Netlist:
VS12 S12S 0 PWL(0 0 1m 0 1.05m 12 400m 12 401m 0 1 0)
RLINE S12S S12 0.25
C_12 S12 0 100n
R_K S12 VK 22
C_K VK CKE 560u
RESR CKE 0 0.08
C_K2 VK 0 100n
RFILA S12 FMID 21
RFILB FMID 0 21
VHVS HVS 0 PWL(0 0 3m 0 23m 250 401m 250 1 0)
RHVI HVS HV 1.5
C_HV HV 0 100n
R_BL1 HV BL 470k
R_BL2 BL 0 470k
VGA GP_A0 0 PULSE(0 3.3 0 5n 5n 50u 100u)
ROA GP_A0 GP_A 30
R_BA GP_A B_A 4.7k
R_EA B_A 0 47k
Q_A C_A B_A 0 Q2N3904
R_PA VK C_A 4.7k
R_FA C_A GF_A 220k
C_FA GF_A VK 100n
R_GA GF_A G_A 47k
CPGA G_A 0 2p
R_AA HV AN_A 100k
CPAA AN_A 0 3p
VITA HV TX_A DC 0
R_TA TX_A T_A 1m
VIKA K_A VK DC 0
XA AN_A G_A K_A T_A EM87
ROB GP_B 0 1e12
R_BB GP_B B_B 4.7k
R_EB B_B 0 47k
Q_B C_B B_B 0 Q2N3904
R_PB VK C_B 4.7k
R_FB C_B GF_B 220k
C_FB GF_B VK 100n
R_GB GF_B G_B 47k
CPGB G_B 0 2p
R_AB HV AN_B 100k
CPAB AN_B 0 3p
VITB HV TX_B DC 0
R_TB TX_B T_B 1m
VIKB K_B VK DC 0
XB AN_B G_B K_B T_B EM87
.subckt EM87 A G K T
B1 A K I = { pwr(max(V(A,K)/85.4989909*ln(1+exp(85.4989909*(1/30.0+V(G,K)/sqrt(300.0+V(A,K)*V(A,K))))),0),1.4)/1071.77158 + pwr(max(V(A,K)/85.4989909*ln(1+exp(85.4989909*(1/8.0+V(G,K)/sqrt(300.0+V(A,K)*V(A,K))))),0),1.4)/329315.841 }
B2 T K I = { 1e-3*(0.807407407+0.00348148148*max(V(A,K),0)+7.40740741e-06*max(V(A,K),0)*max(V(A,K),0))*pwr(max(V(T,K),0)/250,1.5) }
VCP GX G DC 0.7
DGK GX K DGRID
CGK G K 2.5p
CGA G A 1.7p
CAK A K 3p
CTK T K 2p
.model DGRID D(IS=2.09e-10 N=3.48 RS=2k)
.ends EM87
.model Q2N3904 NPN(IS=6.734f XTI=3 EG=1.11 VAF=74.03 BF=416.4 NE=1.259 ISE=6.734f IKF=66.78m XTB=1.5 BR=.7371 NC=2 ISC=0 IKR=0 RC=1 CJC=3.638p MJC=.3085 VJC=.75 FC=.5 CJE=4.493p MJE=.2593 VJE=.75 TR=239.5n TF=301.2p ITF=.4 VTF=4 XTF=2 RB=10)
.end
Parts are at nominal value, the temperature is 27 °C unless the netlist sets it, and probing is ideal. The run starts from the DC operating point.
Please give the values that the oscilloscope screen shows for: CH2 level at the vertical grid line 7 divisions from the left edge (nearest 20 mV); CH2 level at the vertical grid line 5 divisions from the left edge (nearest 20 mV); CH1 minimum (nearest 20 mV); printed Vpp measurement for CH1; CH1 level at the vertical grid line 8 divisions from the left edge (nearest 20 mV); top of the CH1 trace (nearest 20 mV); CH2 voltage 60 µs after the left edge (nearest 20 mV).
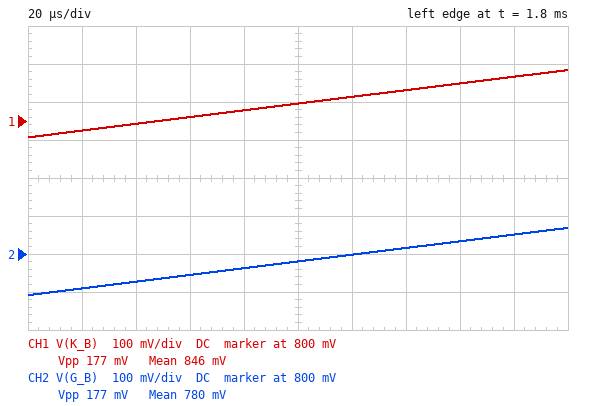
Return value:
820 mV
780 mV
760 mV
177 mV
900 mV
940 mV
740 mV
